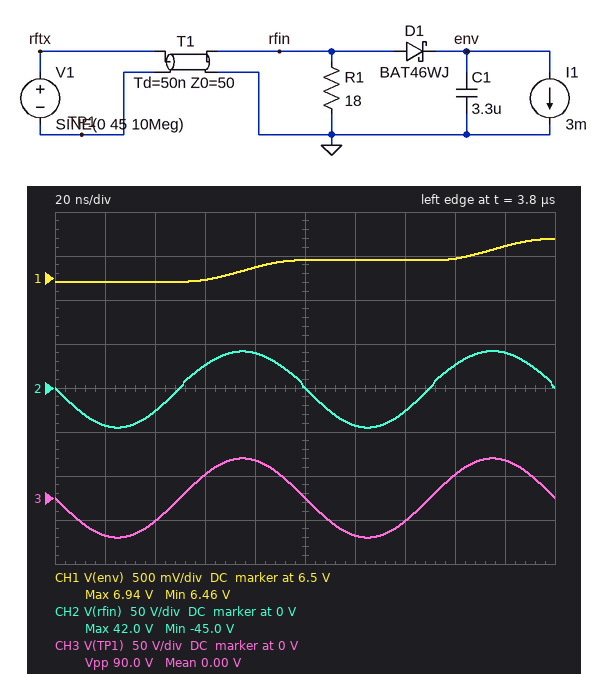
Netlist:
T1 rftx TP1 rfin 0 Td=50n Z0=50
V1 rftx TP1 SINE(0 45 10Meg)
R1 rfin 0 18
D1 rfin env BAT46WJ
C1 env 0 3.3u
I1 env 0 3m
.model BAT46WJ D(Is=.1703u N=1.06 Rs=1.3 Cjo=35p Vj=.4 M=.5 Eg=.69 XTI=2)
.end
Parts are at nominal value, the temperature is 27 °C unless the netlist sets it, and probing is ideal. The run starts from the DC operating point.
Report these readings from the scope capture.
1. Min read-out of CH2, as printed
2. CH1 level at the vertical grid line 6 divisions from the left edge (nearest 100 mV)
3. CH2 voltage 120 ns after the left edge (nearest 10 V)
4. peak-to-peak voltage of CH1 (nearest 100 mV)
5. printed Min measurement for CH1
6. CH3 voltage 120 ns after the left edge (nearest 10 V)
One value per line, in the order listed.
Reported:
-45.0 V
6.7 V
-40 V
500 mV
6.46 V
-40 V
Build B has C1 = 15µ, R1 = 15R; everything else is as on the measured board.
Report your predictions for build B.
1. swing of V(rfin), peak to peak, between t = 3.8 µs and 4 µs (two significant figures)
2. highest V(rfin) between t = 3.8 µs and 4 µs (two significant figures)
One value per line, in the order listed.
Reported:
84 V
39 V
